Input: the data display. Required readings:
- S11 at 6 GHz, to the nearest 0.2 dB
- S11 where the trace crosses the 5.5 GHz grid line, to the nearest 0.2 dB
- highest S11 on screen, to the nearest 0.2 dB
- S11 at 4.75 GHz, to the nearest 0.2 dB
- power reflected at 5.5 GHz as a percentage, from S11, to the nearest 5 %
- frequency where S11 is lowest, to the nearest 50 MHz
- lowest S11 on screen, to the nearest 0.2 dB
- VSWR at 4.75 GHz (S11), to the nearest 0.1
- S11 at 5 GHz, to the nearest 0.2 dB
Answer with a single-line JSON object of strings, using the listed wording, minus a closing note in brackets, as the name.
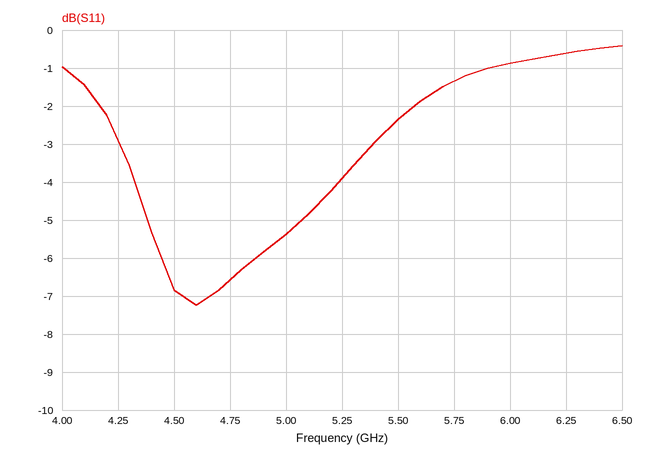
{"S11 at 6 GHz, to the nearest 0.2 dB": "-0.8 dB", "S11 where the trace crosses the 5.5 GHz grid line, to the nearest 0.2 dB": "-2.4 dB", "highest S11 on screen, to the nearest 0.2 dB": "-0.4 dB", "S11 at 4.75 GHz, to the nearest 0.2 dB": "-6.6 dB", "power reflected at 5.5 GHz as a percentage, from S11, to the nearest 5 %": "60 %", "frequency where S11 is lowest, to the nearest 50 MHz": "4.60 GHz", "lowest S11 on screen, to the nearest 0.2 dB": "-7.2 dB", "VSWR at 4.75 GHz (S11), to the nearest 0.1": "2.8", "S11 at 5 GHz, to the nearest 0.2 dB": "-5.4 dB"}
